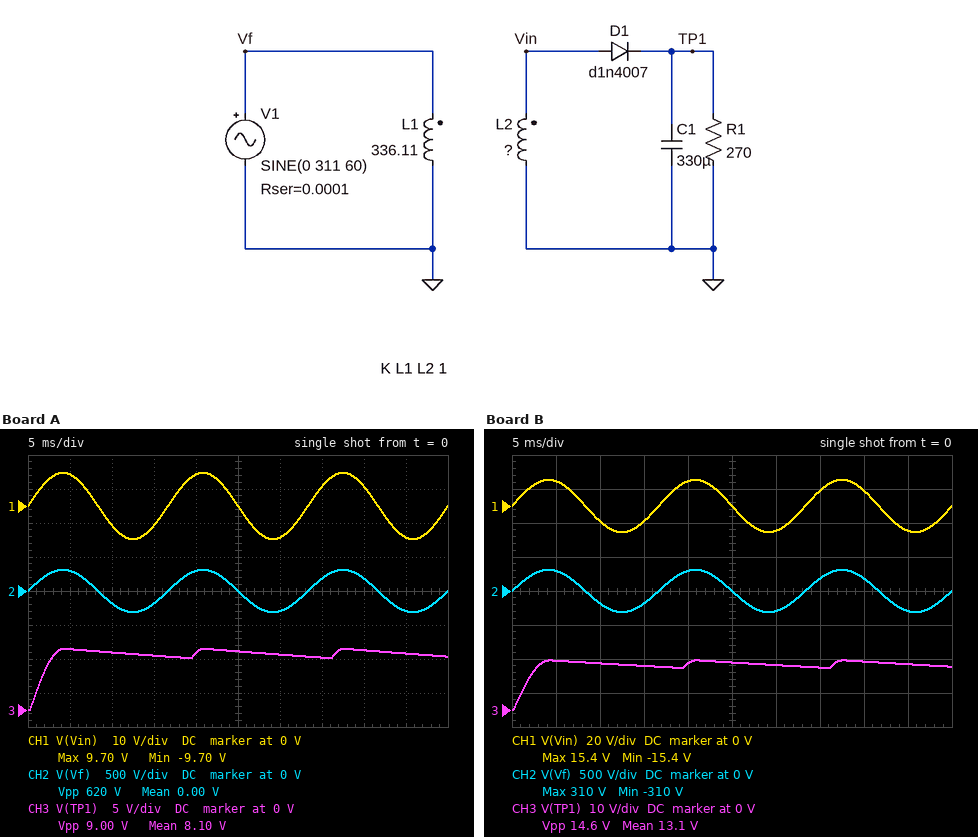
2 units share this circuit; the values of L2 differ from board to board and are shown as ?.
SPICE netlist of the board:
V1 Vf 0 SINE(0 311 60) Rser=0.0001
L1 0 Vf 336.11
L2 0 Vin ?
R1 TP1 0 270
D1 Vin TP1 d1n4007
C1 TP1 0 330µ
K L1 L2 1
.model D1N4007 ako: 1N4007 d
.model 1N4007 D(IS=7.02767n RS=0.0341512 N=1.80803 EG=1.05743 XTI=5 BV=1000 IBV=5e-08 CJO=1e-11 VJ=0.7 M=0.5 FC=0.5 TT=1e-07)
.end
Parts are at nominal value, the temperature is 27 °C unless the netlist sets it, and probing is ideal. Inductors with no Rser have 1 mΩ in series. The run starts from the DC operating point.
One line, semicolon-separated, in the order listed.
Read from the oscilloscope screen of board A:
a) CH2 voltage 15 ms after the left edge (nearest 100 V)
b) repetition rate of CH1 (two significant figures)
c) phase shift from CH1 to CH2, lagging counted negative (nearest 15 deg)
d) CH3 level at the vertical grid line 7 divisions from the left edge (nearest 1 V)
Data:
-200 V; 60 Hz; 0 deg; 8 V
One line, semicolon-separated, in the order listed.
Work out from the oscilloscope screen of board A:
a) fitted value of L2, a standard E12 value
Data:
330 mH
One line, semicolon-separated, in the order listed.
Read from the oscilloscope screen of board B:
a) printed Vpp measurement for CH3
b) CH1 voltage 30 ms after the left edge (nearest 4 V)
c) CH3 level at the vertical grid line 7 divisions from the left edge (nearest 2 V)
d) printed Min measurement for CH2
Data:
14.6 V; -16 V; 12 V; -310 V
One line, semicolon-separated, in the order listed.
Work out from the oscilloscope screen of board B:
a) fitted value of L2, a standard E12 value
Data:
820 mH
